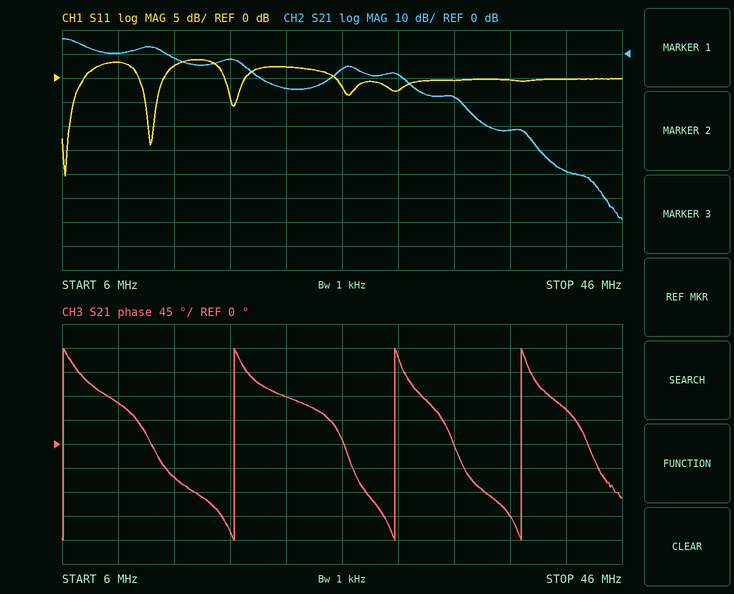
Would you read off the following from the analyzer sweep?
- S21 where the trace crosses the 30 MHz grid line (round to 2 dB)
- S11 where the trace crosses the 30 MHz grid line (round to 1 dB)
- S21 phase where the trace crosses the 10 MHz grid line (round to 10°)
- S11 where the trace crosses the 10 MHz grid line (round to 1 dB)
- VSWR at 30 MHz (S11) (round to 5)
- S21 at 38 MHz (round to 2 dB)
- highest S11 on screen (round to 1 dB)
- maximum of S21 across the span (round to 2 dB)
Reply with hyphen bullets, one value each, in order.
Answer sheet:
- -8 dB
- -3 dB
- 80°
- 3 dB
- 5
- -32 dB
- 4 dB
- 6 dB
